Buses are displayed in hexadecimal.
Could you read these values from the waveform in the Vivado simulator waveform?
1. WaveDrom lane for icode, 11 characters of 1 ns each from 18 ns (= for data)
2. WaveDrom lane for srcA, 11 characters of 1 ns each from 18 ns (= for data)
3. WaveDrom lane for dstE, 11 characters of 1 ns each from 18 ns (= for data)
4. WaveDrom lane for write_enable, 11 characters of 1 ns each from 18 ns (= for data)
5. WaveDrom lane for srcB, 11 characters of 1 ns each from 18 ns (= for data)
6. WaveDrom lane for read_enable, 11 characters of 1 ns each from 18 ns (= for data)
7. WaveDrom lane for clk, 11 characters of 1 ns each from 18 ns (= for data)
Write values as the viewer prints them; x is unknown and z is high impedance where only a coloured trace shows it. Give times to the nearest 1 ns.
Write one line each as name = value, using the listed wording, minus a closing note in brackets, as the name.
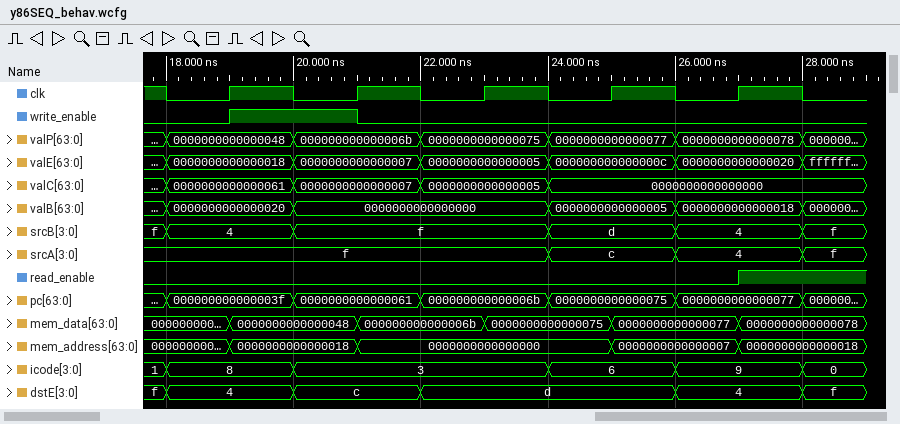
WaveDrom lane for icode, 11 characters of 1 ns each from 18 ns = {name: 'icode', wave: '=.=...=.=.=', data: '8 3 6 9 0'}
WaveDrom lane for srcA, 11 characters of 1 ns each from 18 ns = {name: 'srcA', wave: '=.....=.=.=', data: 'f c 4 f'}
WaveDrom lane for dstE, 11 characters of 1 ns each from 18 ns = {name: 'dstE', wave: '=.=.=...=.=', data: '4 c d 4 f'}
WaveDrom lane for write_enable, 11 characters of 1 ns each from 18 ns = {name: 'write_enable', wave: '01.0.......'}
WaveDrom lane for srcB, 11 characters of 1 ns each from 18 ns = {name: 'srcB', wave: '=.=...=.=.=', data: '4 f d 4 f'}
WaveDrom lane for read_enable, 11 characters of 1 ns each from 18 ns = {name: 'read_enable', wave: '0........1.'}
WaveDrom lane for clk, 11 characters of 1 ns each from 18 ns = {name: 'clk', wave: '01010101010'}
